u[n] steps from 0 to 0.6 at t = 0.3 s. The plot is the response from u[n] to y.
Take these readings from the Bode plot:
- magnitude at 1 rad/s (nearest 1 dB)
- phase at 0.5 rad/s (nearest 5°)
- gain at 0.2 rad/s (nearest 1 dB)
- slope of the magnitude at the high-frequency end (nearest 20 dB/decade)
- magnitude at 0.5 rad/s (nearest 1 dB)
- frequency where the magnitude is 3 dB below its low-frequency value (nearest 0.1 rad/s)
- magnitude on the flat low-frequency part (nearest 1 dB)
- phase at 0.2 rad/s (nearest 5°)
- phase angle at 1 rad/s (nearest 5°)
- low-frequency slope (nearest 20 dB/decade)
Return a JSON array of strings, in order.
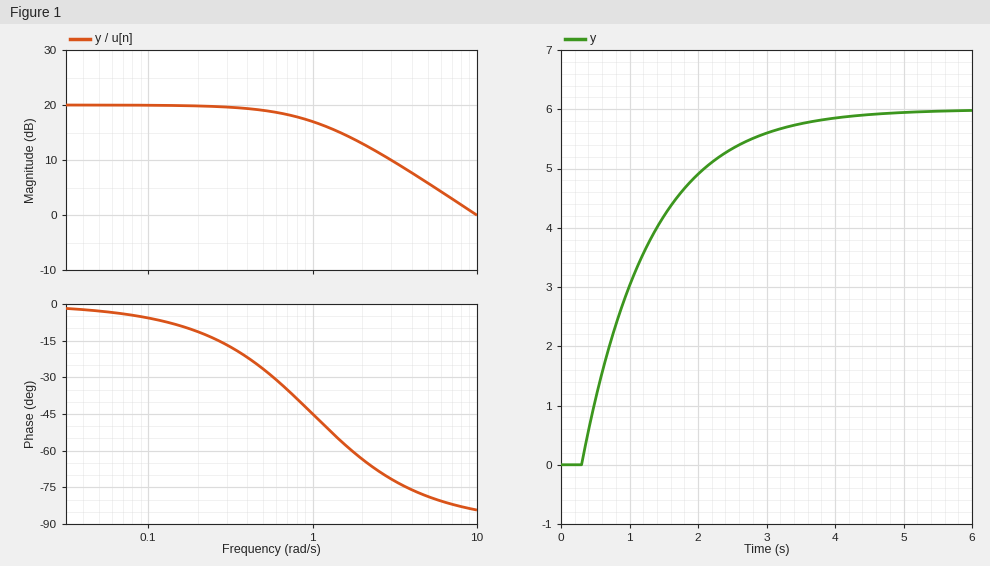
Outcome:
["17 dB", "-25°", "20 dB", "-20 dB/decade", "19 dB", "1.0 rad/s", "20 dB", "-10°", "-45°", "0 dB/decade"]
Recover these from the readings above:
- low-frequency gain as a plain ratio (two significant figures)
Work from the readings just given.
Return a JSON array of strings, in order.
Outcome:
["10"]
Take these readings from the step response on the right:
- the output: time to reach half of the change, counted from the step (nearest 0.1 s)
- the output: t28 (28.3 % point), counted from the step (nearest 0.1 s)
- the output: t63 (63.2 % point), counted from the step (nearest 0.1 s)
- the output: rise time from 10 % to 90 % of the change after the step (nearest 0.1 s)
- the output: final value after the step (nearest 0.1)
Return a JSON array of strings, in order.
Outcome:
["0.7 s", "0.3 s", "1.0 s", "2.2 s", "6.0"]
